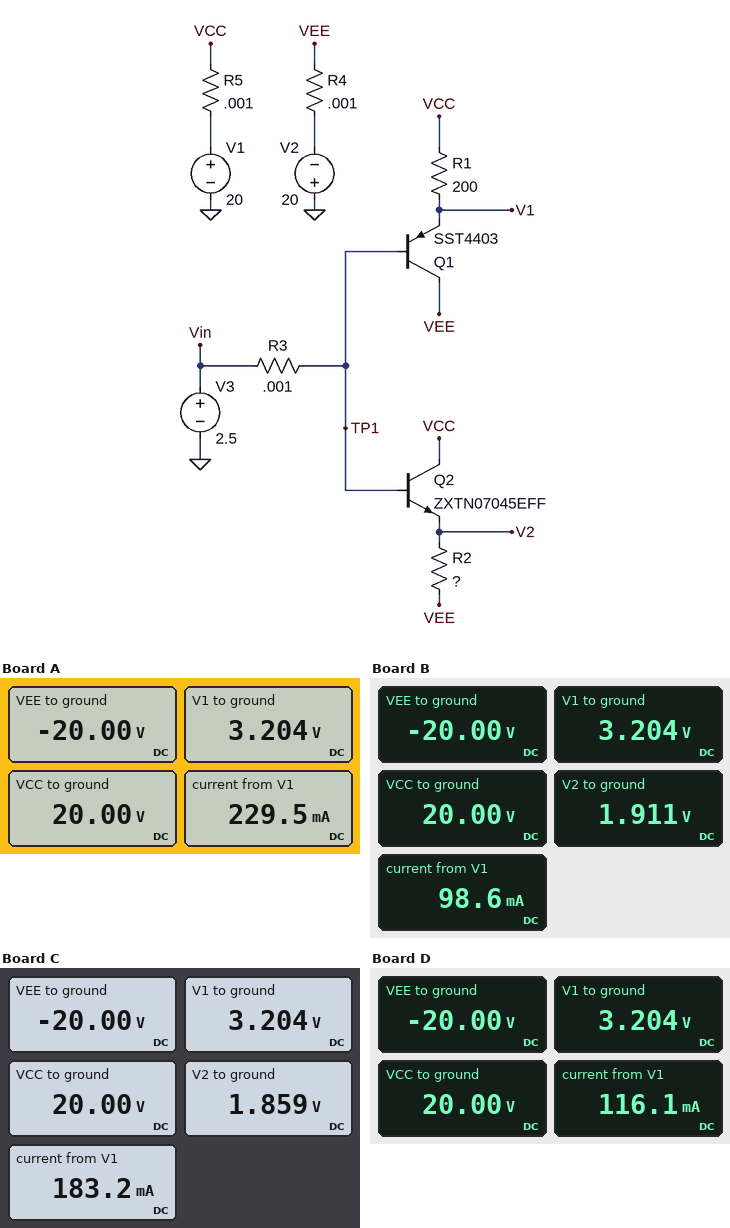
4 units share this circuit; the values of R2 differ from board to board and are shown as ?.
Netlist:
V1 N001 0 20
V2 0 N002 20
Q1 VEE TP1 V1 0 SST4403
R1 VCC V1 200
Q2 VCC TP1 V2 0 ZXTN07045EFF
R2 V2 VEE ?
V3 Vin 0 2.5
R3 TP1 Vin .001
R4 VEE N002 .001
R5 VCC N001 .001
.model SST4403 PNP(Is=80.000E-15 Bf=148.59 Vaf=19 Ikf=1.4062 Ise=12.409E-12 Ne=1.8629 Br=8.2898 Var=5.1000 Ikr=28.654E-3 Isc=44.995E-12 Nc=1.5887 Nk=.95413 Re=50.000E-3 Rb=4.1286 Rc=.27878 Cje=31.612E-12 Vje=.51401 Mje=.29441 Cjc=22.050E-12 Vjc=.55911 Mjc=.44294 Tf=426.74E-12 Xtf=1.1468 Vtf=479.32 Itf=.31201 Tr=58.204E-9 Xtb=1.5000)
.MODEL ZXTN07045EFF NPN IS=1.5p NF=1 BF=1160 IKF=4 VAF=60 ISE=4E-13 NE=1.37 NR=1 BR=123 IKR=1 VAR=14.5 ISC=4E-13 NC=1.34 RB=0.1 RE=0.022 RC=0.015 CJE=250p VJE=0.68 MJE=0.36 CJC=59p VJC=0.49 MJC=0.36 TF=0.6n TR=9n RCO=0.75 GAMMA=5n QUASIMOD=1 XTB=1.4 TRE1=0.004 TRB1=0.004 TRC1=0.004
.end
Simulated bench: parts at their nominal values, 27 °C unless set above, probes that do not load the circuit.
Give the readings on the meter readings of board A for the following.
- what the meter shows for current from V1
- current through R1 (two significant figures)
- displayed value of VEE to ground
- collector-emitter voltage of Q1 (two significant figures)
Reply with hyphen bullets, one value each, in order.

- 229.5 mA
- 84 mA
- -20.00 V
- -23 V
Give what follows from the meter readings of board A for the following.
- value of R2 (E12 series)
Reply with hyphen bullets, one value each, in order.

- 150 Ω
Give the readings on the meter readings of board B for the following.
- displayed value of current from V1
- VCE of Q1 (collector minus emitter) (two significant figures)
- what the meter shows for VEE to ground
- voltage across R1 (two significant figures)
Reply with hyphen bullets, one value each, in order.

- 98.6 mA
- -23 V
- -20.00 V
- 17 V
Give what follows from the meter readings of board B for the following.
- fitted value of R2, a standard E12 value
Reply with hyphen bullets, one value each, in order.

- 1.5 kΩ
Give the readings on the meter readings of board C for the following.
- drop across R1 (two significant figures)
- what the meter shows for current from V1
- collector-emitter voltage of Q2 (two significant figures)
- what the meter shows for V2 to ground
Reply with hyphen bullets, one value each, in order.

- 17 V
- 183.2 mA
- 18 V
- 1.859 V
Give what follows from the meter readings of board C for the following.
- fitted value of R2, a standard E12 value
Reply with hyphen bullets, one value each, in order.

- 220 Ω
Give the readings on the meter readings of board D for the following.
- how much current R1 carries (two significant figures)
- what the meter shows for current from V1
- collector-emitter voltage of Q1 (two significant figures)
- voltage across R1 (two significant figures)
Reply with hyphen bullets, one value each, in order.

- 84 mA
- 116.1 mA
- -23 V
- 17 V
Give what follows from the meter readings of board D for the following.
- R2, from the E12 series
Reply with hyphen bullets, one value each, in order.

- 680 Ω
